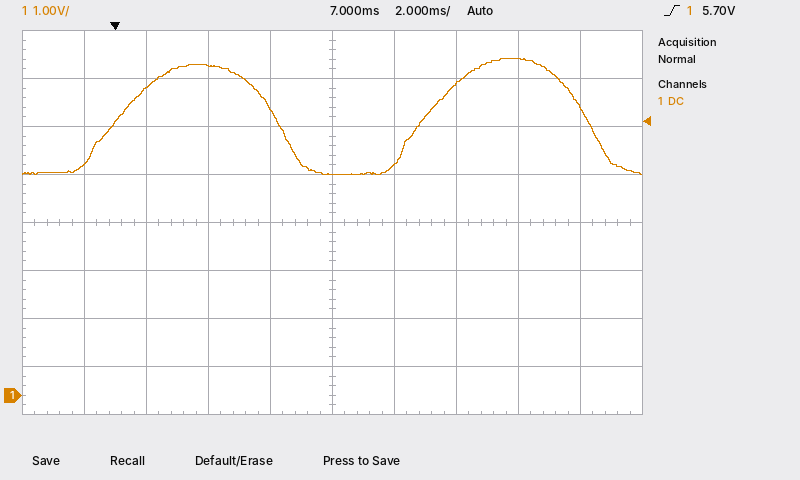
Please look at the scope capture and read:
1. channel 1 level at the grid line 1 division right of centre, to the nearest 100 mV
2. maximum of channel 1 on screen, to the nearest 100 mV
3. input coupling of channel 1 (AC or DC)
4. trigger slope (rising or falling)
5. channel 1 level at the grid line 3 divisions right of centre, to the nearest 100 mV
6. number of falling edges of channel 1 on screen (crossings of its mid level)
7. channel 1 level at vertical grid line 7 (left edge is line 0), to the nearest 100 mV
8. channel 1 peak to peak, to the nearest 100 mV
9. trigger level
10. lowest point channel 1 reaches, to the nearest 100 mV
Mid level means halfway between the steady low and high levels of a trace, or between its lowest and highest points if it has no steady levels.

4.8 V
7.0 V
DC
rising
7.0 V
2
6.5 V
2.4 V
5.70 V
4.6 V
